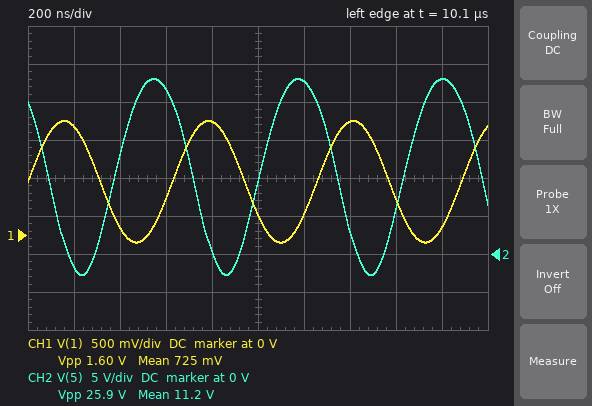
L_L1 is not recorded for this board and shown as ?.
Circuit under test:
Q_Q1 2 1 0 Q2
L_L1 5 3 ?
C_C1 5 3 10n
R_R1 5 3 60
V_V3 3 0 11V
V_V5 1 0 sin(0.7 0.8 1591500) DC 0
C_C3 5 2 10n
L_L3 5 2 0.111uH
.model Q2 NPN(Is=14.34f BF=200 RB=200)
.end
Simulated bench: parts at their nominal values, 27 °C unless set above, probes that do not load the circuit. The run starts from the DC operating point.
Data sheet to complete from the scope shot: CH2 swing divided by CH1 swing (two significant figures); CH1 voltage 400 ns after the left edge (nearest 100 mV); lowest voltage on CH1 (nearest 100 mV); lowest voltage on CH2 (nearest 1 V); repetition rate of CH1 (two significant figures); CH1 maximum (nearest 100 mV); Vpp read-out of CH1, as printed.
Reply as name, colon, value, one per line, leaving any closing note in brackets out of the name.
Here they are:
CH2 swing divided by CH1 swing: 16
CH1 voltage 400 ns after the left edge: 100 mV
lowest voltage on CH1: -100 mV
lowest voltage on CH2: -3 V
repetition rate of CH1: 1.6 MHz
CH1 maximum: 1.5 V
Vpp read-out of CH1, as printed: 1.60 V
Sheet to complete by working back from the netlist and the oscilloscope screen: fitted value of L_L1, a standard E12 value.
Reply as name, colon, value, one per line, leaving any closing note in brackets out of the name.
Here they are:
fitted value of L_L1, a standard E12 value: 1.2 µH
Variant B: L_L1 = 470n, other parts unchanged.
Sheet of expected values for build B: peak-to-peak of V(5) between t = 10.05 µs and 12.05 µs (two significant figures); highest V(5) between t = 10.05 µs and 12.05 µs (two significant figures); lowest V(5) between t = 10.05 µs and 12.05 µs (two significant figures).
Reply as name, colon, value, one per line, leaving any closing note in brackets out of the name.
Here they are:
peak-to-peak of V(5) between t = 10.05 µs and 12.05 µs: 7.9 V
highest V(5) between t = 10.05 µs and 12.05 µs: 15 V
lowest V(5) between t = 10.05 µs and 12.05 µs: 7.4 V
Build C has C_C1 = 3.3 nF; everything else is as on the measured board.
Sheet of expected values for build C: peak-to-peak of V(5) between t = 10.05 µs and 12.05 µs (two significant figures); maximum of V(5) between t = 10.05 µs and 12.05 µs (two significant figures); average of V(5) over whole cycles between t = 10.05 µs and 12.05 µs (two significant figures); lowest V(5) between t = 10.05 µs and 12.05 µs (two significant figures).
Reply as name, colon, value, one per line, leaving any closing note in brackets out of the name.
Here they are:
peak-to-peak of V(5) between t = 10.05 µs and 12.05 µs: 18 V
maximum of V(5) between t = 10.05 µs and 12.05 µs: 22 V
average of V(5) over whole cycles between t = 10.05 µs and 12.05 µs: 11 V
lowest V(5) between t = 10.05 µs and 12.05 µs: 4.2 V
